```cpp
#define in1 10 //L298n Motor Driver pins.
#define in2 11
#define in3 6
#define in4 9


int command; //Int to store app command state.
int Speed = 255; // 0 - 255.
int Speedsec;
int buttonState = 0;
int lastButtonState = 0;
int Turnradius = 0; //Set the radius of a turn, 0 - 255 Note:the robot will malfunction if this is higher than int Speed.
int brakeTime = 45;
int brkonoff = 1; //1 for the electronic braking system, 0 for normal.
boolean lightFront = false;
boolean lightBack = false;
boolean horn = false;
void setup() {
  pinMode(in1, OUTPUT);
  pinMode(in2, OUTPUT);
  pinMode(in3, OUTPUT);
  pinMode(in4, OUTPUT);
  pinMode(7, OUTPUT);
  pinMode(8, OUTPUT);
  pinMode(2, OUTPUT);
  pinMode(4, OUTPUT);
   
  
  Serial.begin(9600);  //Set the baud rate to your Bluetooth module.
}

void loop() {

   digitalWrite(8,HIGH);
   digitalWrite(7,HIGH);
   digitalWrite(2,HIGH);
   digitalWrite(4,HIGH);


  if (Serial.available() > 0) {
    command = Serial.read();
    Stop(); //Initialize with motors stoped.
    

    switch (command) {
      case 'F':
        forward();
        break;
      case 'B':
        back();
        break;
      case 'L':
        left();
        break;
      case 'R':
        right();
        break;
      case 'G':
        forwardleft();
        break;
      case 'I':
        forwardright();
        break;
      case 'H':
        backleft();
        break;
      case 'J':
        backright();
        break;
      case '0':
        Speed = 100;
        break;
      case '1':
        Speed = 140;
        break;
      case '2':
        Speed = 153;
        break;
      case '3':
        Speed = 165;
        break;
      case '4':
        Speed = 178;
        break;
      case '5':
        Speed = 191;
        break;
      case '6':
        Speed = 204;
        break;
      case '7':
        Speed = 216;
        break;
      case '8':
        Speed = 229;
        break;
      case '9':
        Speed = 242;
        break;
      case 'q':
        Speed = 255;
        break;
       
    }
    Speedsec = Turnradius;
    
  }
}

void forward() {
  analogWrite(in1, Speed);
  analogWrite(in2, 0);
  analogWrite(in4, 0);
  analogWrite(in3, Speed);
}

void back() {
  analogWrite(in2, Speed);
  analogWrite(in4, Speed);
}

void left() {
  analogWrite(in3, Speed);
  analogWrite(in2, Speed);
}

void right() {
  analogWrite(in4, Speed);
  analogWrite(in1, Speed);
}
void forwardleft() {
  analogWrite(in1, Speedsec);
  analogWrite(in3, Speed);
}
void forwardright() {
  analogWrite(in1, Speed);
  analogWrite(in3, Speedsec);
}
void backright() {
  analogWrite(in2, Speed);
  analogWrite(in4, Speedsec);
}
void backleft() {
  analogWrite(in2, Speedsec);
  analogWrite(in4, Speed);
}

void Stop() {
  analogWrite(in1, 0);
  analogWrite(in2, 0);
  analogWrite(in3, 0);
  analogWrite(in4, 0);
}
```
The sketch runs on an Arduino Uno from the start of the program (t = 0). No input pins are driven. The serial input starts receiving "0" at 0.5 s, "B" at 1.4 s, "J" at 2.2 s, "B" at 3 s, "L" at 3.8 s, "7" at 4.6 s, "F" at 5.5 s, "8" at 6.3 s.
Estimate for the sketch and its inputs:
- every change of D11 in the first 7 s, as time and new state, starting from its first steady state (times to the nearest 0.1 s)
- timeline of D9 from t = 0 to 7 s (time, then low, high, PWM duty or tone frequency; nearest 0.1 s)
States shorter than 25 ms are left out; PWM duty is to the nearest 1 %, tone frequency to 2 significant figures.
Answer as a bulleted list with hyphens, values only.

- 0 s low; 1.4 s PWM 39 %; 4.6 s low
- 0 s low; 1.4 s PWM 39 %; 2.2 s low; 3 s PWM 39 %; 3.8 s low
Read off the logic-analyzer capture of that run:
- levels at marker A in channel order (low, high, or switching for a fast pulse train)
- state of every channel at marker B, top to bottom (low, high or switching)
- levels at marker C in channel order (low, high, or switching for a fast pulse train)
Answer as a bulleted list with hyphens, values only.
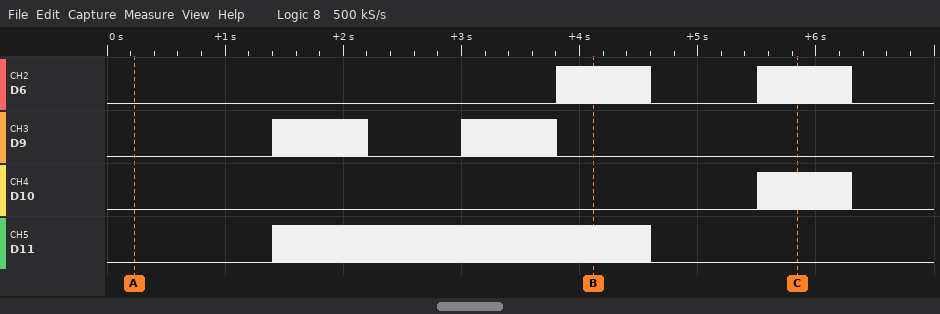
- D6 low, D9 low, D10 low, D11 low
- D6 switching, D9 low, D10 low, D11 switching
- D6 switching, D9 low, D10 switching, D11 low
